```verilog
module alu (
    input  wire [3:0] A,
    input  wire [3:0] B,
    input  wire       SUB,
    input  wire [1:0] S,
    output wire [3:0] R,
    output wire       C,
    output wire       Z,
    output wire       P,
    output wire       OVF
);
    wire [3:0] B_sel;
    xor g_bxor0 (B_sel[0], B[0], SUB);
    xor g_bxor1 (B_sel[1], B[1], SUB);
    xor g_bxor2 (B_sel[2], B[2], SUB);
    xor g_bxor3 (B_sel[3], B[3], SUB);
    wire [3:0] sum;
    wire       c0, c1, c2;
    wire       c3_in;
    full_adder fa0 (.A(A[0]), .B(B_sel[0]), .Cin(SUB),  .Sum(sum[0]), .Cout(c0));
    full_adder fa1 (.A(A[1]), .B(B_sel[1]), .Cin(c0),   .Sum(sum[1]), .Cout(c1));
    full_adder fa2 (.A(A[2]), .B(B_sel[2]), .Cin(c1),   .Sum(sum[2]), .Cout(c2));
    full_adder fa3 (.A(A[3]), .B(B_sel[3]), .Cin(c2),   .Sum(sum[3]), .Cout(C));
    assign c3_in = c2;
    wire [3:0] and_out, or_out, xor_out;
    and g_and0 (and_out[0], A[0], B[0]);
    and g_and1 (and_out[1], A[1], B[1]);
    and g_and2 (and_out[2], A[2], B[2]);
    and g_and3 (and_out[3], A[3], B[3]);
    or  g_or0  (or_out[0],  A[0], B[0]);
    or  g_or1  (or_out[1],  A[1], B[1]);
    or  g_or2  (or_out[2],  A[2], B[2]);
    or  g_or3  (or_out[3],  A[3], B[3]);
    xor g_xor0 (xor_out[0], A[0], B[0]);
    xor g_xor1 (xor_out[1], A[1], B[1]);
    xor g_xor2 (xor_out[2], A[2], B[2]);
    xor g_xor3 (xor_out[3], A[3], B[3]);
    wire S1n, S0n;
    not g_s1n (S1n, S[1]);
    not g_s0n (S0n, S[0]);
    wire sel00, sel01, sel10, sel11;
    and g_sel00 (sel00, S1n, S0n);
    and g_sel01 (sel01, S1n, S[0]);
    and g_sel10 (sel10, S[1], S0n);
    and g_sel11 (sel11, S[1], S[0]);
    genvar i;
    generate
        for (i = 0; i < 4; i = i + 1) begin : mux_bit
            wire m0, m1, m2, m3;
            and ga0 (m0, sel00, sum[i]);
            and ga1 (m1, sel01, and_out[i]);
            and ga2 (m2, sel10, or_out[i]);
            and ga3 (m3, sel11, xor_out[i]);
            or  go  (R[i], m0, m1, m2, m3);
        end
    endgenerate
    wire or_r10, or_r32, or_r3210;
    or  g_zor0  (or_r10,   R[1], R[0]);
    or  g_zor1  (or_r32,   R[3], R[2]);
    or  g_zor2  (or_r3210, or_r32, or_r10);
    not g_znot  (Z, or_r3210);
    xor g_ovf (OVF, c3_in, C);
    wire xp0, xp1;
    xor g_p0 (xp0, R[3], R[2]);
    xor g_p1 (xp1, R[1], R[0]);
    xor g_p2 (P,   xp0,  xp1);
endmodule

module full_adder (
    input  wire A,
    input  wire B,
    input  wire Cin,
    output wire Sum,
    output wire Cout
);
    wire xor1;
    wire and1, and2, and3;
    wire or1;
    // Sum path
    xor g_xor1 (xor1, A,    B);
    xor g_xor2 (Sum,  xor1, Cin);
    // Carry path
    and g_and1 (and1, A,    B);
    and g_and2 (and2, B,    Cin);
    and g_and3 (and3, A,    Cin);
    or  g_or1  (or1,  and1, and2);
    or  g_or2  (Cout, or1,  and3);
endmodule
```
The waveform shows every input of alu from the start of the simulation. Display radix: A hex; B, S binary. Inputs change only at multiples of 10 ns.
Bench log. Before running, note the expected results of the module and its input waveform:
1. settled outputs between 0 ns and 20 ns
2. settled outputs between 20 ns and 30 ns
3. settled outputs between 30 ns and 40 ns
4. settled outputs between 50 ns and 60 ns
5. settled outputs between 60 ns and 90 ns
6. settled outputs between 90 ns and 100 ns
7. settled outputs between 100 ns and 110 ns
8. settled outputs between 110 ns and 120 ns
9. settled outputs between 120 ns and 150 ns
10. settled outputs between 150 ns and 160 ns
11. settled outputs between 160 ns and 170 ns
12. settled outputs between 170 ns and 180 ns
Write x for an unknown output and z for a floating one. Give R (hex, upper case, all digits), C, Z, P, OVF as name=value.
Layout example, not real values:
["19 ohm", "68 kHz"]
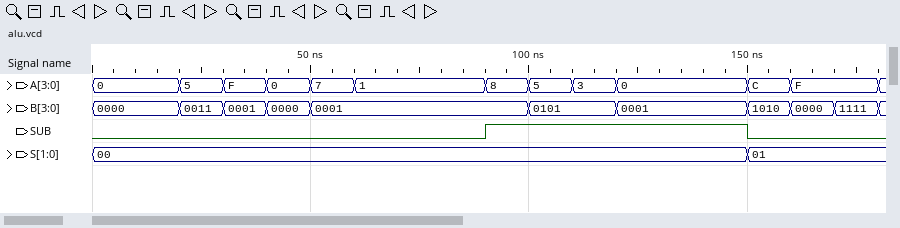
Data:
["R=0, C=0, Z=1, P=0, OVF=0", "R=8, C=0, Z=0, P=1, OVF=1", "R=0, C=1, Z=1, P=0, OVF=0", "R=8, C=0, Z=0, P=1, OVF=1", "R=2, C=0, Z=0, P=1, OVF=0", "R=7, C=1, Z=0, P=1, OVF=1", "R=0, C=1, Z=1, P=0, OVF=0", "R=E, C=0, Z=0, P=1, OVF=0", "R=F, C=0, Z=0, P=0, OVF=0", "R=8, C=1, Z=0, P=1, OVF=1", "R=0, C=0, Z=1, P=0, OVF=0", "R=F, C=1, Z=0, P=0, OVF=0"]
